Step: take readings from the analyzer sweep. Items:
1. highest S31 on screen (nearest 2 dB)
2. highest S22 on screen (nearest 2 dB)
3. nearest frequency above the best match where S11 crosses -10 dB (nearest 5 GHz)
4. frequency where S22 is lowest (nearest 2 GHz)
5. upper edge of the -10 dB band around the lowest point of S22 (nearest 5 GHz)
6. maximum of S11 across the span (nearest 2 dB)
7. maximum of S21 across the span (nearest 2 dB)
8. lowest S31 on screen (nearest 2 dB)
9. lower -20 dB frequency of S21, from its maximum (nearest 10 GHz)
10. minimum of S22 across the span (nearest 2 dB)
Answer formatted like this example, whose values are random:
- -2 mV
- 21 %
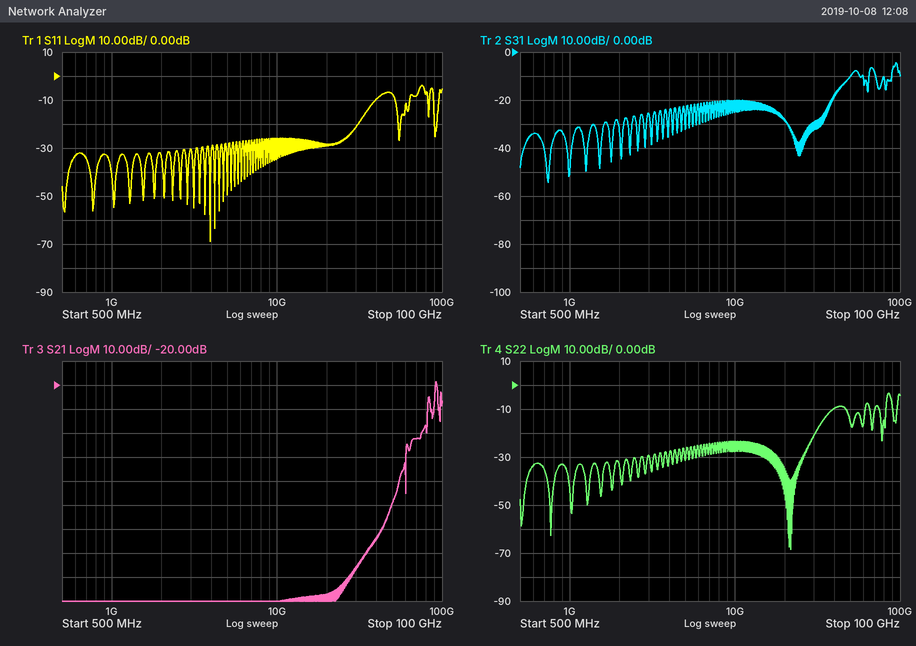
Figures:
- -4 dB
- -4 dB
- 40 GHz
- 22 GHz
- 40 GHz
- -4 dB
- -18 dB
- -54 dB
- 80 GHz
- -68 dB
